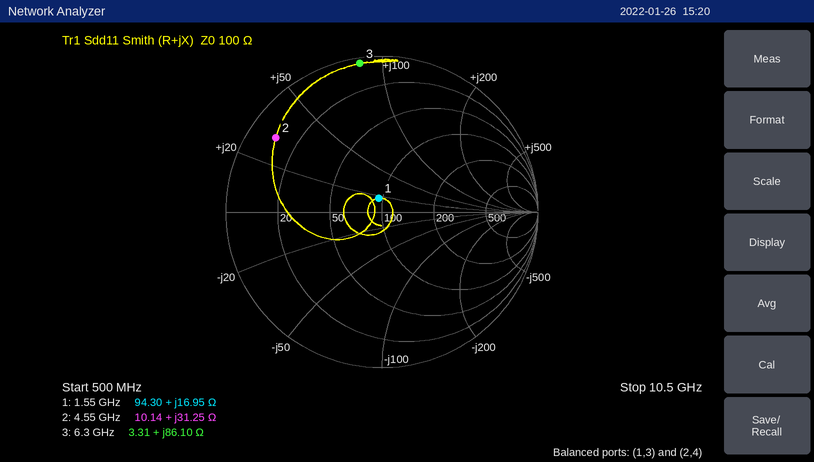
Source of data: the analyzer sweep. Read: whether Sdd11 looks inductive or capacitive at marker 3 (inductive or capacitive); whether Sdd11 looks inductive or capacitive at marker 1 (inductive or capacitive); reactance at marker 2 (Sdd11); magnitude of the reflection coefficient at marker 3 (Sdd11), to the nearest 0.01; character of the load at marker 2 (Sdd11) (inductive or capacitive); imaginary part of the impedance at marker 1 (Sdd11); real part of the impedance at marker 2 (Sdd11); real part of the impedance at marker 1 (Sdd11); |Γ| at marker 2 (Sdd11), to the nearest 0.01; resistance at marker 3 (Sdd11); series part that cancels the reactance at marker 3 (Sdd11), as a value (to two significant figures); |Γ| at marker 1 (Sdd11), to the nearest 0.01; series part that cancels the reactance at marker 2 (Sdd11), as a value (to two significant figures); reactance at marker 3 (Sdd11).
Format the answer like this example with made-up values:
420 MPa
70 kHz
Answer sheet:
inductive
inductive
+31.25 Ω
0.96
inductive
+16.95 Ω
10.14 Ω
94.30 Ω
0.83
3.31 Ω
290 fF
0.09
1.1 pF
+86.10 Ω
